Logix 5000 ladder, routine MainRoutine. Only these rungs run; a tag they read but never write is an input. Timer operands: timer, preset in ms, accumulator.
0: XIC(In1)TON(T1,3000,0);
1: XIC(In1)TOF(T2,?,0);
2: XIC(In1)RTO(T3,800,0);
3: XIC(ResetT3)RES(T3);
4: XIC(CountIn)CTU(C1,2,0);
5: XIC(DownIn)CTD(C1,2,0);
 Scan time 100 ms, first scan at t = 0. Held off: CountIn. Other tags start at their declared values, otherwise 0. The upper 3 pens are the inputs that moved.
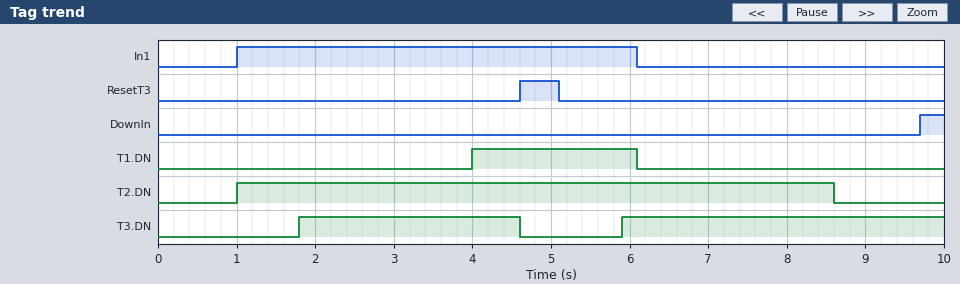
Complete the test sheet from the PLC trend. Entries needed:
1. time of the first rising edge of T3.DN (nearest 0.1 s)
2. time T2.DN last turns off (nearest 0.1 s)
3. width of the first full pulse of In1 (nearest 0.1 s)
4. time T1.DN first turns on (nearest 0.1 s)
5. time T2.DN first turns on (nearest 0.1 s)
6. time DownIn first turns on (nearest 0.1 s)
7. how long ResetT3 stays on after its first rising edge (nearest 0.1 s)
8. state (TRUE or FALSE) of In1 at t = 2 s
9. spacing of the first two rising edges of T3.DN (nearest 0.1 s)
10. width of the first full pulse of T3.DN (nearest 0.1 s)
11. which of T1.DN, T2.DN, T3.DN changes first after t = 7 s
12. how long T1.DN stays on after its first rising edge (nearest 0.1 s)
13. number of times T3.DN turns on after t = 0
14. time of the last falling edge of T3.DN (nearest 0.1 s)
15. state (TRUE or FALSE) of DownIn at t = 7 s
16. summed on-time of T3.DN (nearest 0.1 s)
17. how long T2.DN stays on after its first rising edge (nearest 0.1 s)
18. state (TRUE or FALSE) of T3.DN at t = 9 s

1.8 s
8.6 s
5.1 s
4.0 s
1.0 s
9.7 s
0.5 s
TRUE
4.1 s
2.8 s
T2.DN
2.1 s
2
4.6 s
FALSE
6.9 s
7.6 s
TRUE
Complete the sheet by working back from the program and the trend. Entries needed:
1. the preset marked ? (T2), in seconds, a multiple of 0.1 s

2.5 s
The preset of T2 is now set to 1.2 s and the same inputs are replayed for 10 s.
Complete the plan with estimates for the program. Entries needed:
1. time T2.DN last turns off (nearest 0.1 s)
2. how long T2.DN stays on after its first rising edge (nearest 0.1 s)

7.3 s
6.3 s
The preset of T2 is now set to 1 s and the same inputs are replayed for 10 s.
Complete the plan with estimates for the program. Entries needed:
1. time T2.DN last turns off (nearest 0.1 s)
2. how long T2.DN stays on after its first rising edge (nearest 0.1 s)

7.1 s
6.1 s
